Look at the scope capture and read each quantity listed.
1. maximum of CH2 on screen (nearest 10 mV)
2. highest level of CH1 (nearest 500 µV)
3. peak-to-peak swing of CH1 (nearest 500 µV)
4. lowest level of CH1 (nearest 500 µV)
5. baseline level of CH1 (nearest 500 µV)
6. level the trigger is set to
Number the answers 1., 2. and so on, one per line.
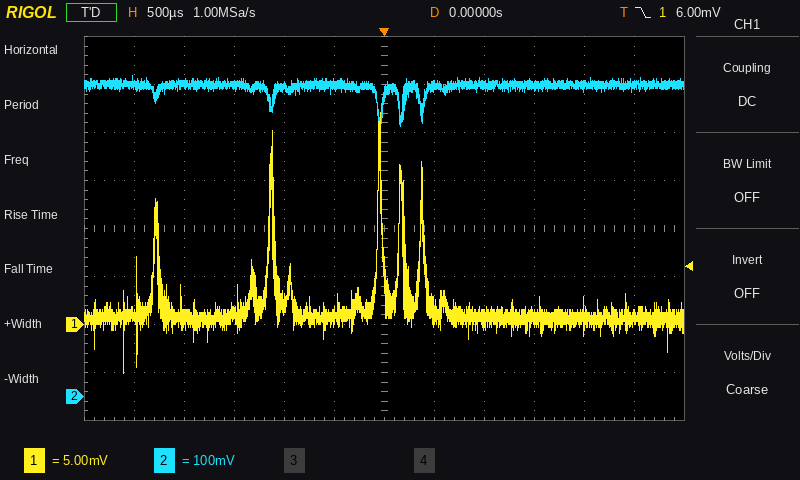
1. 670 mV
2. 22.0 mV
3. 27.0 mV
4. -5.0 mV
5. 1.0 mV
6. 6.00 mV
